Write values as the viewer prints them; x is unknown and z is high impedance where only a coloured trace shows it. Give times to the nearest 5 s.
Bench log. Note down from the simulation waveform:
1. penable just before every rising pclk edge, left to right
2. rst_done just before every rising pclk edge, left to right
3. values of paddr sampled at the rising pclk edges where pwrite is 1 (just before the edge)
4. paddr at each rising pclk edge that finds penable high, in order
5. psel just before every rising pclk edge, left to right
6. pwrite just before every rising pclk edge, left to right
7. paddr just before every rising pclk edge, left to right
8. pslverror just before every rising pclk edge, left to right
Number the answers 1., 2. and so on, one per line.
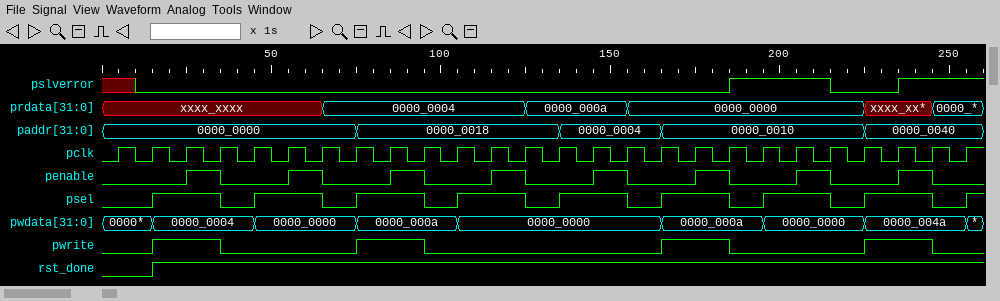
1. 0 0 0 1 0 0 1 0 0 1 0 0 1 0 0 1 0 0 1 0 0 1 0 0 1 0
2. 0 0 1 1 1 1 1 1 1 1 1 1 1 1 1 1 1 1 1 1 1 1 1 1 1 1
3. 0000_0000, 0000_0000, 0000_0018, 0000_0018, 0000_0010, 0000_0010, 0000_0040, 0000_0040
4. 0000_0000, 0000_0000, 0000_0018, 0000_0018, 0000_0004, 0000_0010, 0000_0010, 0000_0040
5. 0 0 1 1 0 1 1 0 1 1 0 1 1 0 1 1 0 1 1 0 1 1 0 1 1 0
6. 0 0 1 1 0 0 0 0 1 1 0 0 0 0 0 0 0 1 1 0 0 0 0 1 1 0
7. 0000_0000, 0000_0000, 0000_0000, 0000_0000, 0000_0000, 0000_0000, 0000_0000, 0000_0000, 0000_0018, 0000_0018, 0000_0018, 0000_0018, 0000_0018, 0000_0018, 0000_0004, 0000_0004, 0000_0004, 0000_0010, 0000_0010, 0000_0010, 0000_0010, 0000_0010, 0000_0010, 0000_0040, 0000_0040, 0000_0040
8. x 0 0 0 0 0 0 0 0 0 0 0 0 0 0 0 0 0 0 1 1 1 0 0 1 1
